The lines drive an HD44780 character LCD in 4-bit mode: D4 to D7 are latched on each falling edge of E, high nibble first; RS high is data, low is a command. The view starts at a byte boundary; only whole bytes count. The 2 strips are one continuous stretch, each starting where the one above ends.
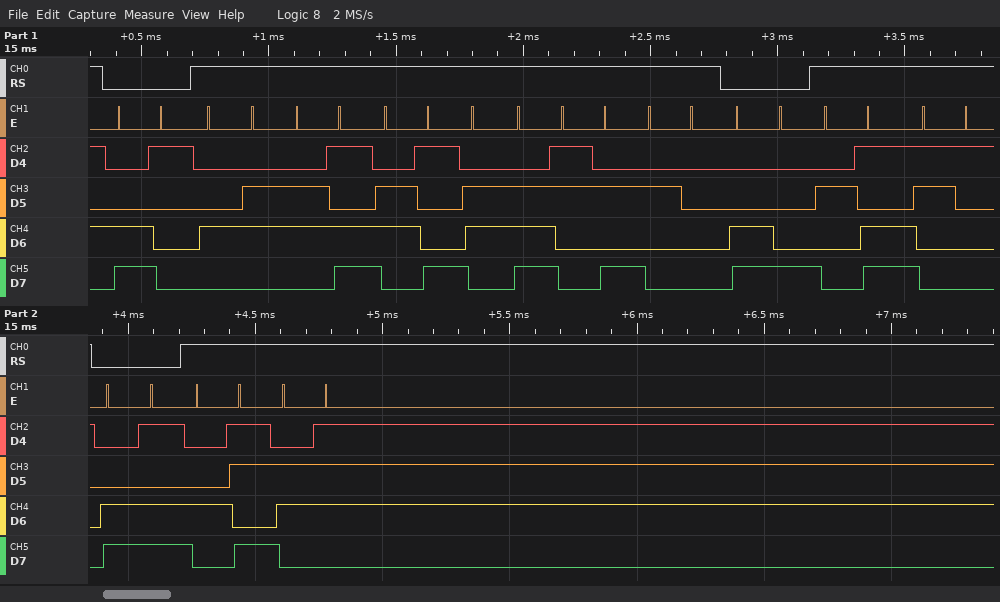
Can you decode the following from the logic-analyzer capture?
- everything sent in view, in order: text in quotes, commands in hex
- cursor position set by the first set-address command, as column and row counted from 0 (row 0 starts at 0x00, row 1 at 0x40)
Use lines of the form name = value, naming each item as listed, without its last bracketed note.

everything sent in view, in order: text in quotes, commands in hex = 0xC1 "Fmin: " 0xC8 "-1" 0xCD "Kg"
cursor position set by the first set-address command, as column and row counted from 0 = column 1, row 1
